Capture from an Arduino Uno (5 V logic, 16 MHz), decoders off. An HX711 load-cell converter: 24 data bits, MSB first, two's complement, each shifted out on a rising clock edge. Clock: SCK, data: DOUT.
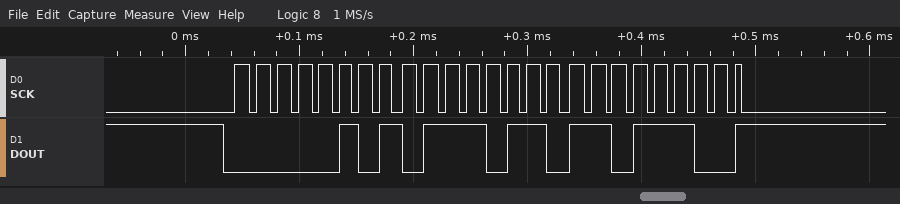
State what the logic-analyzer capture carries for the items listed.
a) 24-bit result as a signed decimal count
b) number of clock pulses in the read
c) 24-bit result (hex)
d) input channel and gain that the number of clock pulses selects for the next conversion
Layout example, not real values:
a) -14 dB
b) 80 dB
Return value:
a) 358108
b) 25
c) 0x0576DC
d) channel A, gain 128
